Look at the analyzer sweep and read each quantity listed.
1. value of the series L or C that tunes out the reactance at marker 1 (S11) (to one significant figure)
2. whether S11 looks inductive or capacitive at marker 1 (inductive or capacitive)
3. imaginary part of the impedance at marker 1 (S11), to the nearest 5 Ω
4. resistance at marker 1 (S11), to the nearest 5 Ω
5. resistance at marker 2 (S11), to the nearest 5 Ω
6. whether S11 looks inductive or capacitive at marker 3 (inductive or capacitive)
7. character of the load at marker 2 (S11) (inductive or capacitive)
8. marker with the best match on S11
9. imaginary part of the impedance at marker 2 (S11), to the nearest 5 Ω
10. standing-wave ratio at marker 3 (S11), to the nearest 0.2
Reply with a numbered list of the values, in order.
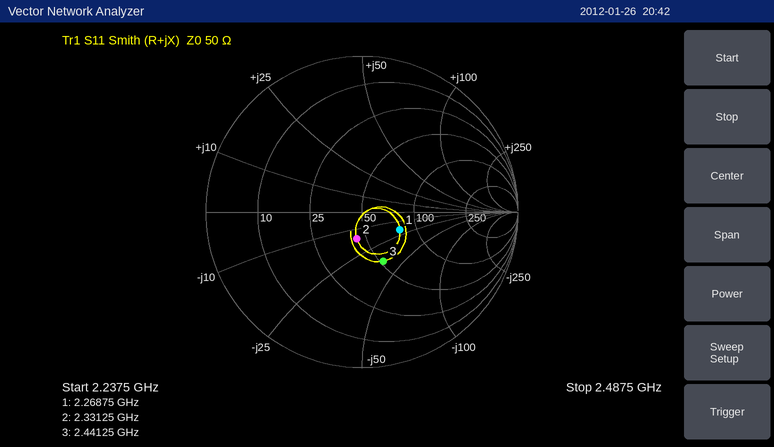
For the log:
1. 1 nH
2. capacitive
3. -20 Ω
4. 80 Ω
5. 45 Ω
6. capacitive
7. capacitive
8. marker 2
9. -15 Ω
10. 2.0
